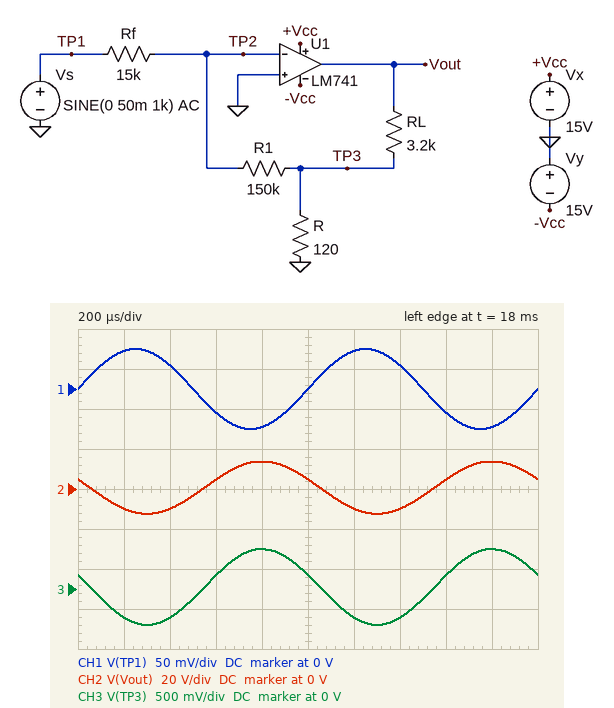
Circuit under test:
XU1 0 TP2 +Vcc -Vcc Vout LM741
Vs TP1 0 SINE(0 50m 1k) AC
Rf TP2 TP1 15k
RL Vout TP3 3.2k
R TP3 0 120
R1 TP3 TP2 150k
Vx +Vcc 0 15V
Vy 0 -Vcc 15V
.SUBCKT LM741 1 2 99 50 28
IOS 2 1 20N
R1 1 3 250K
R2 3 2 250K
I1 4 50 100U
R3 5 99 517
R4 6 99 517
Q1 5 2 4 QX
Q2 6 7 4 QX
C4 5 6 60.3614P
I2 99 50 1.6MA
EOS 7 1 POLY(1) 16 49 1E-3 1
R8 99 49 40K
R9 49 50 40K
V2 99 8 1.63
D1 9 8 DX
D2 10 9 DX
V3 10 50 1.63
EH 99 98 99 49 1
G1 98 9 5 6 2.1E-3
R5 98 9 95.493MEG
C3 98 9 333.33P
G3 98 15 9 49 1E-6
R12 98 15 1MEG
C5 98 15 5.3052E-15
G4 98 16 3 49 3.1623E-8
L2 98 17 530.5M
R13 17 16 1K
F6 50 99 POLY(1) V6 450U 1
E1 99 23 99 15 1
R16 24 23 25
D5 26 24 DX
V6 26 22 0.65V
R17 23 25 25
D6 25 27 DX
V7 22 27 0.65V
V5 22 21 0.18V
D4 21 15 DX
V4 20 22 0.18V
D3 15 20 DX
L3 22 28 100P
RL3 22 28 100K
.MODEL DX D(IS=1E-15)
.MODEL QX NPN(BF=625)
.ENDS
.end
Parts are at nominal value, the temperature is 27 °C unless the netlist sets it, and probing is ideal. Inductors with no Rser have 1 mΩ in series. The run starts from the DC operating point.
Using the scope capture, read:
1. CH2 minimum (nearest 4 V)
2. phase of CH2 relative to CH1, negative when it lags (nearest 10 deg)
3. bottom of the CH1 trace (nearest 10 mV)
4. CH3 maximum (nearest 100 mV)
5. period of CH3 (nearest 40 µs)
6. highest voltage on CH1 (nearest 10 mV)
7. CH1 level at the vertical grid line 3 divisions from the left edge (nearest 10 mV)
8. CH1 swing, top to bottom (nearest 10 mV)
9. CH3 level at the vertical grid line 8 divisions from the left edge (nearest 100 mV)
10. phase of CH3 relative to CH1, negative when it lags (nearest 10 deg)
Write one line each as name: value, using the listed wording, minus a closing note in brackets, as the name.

CH2 minimum: -12 V
phase of CH2 relative to CH1, negative when it lags: 160 deg
bottom of the CH1 trace: -50 mV
CH3 maximum: 500 mV
period of CH3: 1.00 ms
highest voltage on CH1: 50 mV
CH1 level at the vertical grid line 3 divisions from the left edge: -30 mV
CH1 swing, top to bottom: 100 mV
CH3 level at the vertical grid line 8 divisions from the left edge: 200 mV
phase of CH3 relative to CH1, negative when it lags: 160 deg
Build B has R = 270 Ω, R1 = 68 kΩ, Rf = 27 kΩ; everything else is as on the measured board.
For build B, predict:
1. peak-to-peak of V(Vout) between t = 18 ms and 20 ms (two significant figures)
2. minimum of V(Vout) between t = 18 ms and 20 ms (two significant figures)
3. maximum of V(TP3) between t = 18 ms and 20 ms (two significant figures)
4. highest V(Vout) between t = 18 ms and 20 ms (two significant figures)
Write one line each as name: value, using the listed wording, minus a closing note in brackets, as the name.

peak-to-peak of V(Vout) between t = 18 ms and 20 ms: 3.2 V
minimum of V(Vout) between t = 18 ms and 20 ms: -1.5 V
maximum of V(TP3) between t = 18 ms and 20 ms: 140 mV
highest V(Vout) between t = 18 ms and 20 ms: 1.8 V
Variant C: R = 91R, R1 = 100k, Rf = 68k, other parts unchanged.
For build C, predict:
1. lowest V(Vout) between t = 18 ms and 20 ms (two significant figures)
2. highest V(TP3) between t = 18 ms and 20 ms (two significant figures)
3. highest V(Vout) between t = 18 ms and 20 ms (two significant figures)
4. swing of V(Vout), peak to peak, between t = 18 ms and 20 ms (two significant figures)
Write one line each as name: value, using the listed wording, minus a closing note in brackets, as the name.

lowest V(Vout) between t = 18 ms and 20 ms: -2.2 V
highest V(TP3) between t = 18 ms and 20 ms: 86 mV
highest V(Vout) between t = 18 ms and 20 ms: 3.1 V
swing of V(Vout), peak to peak, between t = 18 ms and 20 ms: 5.3 V
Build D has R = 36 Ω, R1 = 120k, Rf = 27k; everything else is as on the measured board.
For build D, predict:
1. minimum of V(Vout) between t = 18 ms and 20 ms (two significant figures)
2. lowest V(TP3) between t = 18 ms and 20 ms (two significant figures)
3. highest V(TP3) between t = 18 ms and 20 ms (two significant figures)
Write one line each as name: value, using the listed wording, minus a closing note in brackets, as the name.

minimum of V(Vout) between t = 18 ms and 20 ms: -14 V
lowest V(TP3) between t = 18 ms and 20 ms: -150 mV
highest V(TP3) between t = 18 ms and 20 ms: 150 mV
